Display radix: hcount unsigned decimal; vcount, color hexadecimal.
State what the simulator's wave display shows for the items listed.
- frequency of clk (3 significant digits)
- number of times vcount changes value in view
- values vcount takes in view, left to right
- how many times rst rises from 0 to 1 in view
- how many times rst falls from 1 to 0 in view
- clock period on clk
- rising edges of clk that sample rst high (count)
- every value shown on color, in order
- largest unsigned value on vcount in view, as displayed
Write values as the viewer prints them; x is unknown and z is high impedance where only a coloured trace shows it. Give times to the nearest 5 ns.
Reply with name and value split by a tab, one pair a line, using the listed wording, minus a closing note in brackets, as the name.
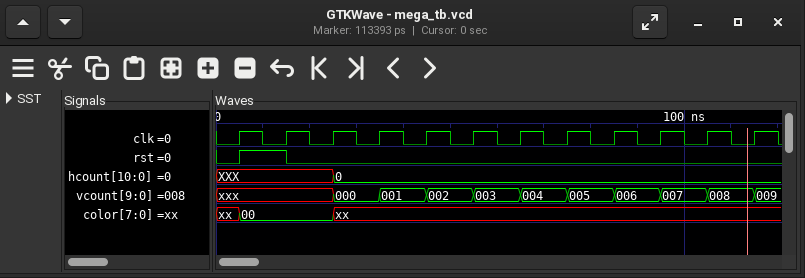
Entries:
frequency of clk	100 MHz
number of times vcount changes value in view	10
values vcount takes in view, left to right	xxx, 000, 001, 002, 003, 004, 005, 006, 007, 008, 009
how many times rst rises from 0 to 1 in view	1
how many times rst falls from 1 to 0 in view	1
clock period on clk	10 ns
rising edges of clk that sample rst high	1
every value shown on color, in order	xx, 00, xx
largest unsigned value on vcount in view, as displayed	009
